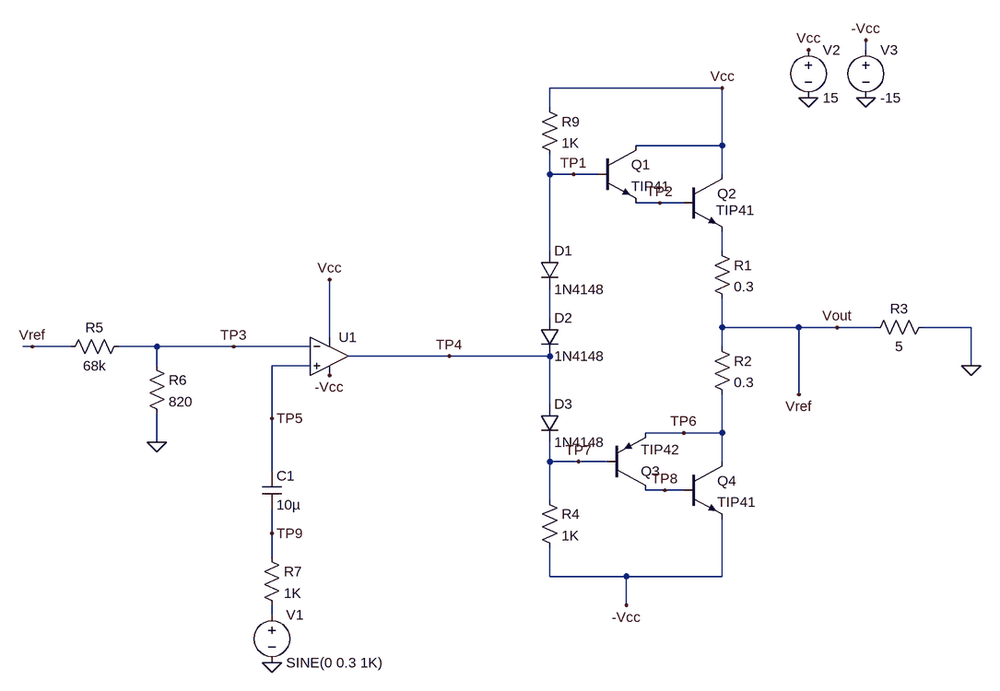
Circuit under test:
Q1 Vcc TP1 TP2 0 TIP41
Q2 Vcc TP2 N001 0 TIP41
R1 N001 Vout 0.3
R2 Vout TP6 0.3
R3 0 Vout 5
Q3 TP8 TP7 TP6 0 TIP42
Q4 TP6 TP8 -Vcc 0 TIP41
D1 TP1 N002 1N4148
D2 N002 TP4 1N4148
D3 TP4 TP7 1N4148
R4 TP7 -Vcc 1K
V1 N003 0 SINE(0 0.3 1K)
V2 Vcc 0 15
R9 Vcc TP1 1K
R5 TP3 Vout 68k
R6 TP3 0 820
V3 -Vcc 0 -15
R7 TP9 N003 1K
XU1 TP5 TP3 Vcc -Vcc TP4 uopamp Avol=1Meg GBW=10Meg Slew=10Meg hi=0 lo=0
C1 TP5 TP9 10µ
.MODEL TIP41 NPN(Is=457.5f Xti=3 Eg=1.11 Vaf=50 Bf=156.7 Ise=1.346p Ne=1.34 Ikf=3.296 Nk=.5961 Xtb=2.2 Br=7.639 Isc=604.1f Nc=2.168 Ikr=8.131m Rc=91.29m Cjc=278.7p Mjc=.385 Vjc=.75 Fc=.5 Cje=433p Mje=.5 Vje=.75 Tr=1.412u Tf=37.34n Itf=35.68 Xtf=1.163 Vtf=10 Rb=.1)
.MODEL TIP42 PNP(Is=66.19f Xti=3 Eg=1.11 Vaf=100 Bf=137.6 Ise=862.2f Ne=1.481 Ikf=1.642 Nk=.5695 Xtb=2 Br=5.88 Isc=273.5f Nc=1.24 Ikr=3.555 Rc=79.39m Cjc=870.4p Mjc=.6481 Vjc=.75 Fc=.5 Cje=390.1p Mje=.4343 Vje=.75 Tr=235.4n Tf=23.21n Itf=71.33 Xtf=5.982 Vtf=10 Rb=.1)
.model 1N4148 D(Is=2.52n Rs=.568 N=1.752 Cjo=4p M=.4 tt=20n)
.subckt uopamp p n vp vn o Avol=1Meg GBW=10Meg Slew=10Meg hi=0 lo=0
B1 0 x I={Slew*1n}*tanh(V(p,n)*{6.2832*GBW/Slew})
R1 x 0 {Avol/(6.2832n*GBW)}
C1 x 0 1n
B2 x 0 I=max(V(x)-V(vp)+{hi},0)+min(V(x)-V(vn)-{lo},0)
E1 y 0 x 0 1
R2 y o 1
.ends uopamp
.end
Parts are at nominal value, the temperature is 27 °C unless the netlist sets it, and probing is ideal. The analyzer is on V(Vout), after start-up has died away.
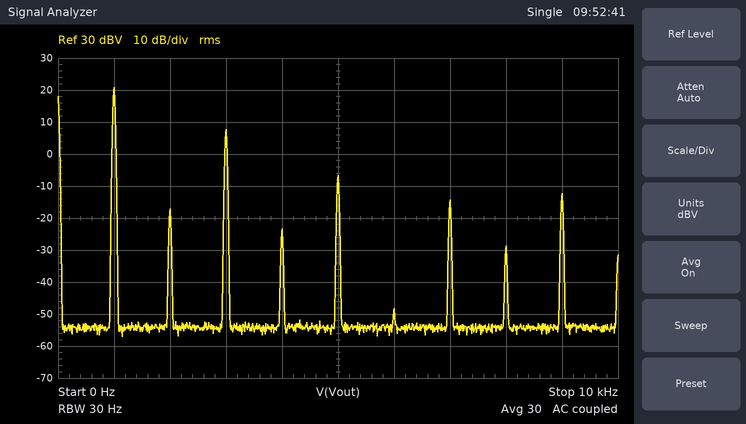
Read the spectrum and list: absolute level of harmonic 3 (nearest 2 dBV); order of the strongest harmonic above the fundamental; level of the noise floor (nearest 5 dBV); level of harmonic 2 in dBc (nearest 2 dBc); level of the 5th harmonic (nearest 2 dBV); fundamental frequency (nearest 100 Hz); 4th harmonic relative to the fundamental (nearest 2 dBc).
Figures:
8 dBV
3
-55 dBV
-38 dBc
-6 dBV
1.0 kHz
-44 dBc
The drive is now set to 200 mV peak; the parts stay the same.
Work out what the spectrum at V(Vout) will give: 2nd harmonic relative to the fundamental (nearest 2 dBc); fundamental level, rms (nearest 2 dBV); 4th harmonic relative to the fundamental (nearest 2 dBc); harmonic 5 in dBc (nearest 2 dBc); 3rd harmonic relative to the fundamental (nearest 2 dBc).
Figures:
-36 dBc
20 dBV
-52 dBc
-30 dBc
-20 dBc
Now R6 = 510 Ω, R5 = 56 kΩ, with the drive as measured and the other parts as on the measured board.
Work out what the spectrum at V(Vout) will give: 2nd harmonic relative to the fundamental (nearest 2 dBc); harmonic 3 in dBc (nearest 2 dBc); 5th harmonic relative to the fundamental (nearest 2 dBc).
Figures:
-40 dBc
-12 dBc
-20 dBc
